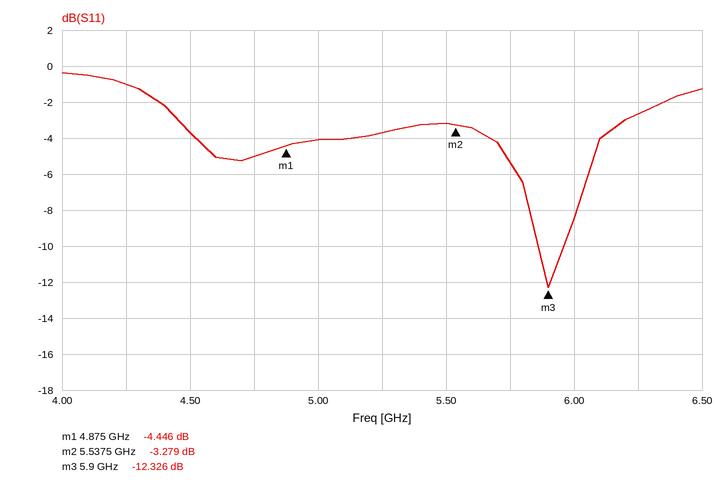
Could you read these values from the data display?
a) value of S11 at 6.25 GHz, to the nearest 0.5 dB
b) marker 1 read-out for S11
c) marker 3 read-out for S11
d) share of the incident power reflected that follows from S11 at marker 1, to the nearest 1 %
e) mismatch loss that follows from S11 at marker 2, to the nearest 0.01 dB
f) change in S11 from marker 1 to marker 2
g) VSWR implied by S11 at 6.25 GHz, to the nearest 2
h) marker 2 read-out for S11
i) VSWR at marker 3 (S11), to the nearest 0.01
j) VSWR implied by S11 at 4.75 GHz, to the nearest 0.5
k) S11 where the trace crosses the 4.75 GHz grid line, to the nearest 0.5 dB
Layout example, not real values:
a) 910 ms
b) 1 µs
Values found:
a) -2.5 dB
b) -4.446 dB
c) -12.326 dB
d) 36 %
e) 2.76 dB
f) 1.167 dB
g) 6
h) -3.279 dB
i) 1.64
j) 3.5
k) -5.0 dB
